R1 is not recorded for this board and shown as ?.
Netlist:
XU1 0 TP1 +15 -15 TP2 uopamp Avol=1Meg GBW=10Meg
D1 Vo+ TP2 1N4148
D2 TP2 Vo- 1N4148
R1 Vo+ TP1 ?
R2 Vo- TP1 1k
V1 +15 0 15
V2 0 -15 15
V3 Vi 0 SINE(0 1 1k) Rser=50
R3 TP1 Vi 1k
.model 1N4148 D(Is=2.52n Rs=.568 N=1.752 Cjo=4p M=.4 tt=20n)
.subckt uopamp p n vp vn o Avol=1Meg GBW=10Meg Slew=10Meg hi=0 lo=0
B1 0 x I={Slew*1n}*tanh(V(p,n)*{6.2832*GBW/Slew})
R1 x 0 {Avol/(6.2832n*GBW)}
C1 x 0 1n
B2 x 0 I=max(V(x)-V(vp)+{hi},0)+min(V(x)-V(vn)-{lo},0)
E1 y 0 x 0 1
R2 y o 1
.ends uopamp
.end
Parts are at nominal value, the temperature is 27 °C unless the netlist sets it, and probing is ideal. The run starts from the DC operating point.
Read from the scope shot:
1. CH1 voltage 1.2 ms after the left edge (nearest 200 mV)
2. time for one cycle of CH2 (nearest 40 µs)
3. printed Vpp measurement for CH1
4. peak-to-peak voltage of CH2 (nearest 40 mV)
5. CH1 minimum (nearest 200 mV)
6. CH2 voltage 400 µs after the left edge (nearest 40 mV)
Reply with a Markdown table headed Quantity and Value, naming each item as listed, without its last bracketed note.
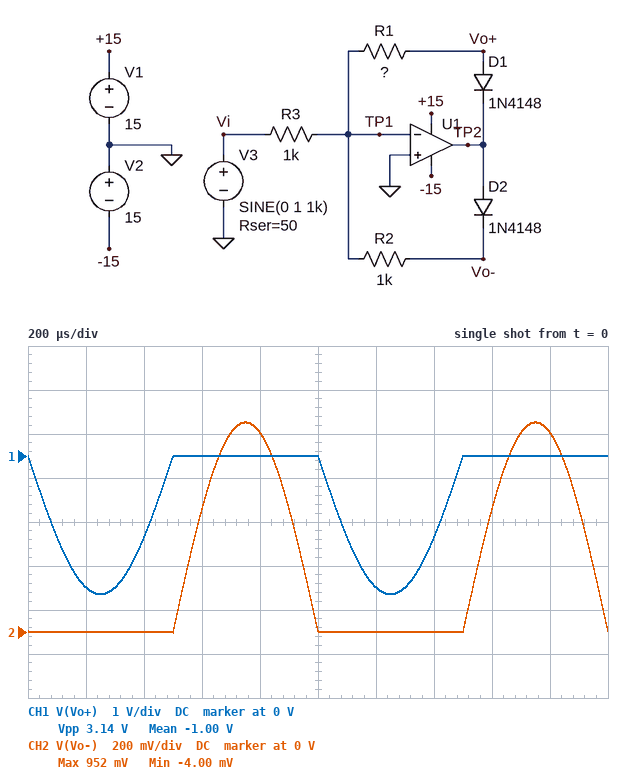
| Quantity | Value |
|---|---|
| CH1 voltage 1.2 ms after the left edge | -3.0 V |
| time for one cycle of CH2 | 1.00 ms |
| printed Vpp measurement for CH1 | 3.14 V |
| peak-to-peak voltage of CH2 | 960 mV |
| CH1 minimum | -3.2 V |
| CH2 voltage 400 µs after the left edge | 0 V |
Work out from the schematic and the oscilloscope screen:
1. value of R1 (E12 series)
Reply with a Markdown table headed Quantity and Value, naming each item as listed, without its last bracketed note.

| Quantity | Value |
|---|---|
| value of R1 | 3.3 kΩ |
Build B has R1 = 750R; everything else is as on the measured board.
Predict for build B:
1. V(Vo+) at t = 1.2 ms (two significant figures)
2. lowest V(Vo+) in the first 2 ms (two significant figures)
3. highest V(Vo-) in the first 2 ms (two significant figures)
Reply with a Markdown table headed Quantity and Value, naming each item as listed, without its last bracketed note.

| Quantity | Value |
|---|---|
| V(Vo+) at t = 1.2 ms | -680 mV |
| lowest V(Vo+) in the first 2 ms | -710 mV |
| highest V(Vo-) in the first 2 ms | 950 mV |
